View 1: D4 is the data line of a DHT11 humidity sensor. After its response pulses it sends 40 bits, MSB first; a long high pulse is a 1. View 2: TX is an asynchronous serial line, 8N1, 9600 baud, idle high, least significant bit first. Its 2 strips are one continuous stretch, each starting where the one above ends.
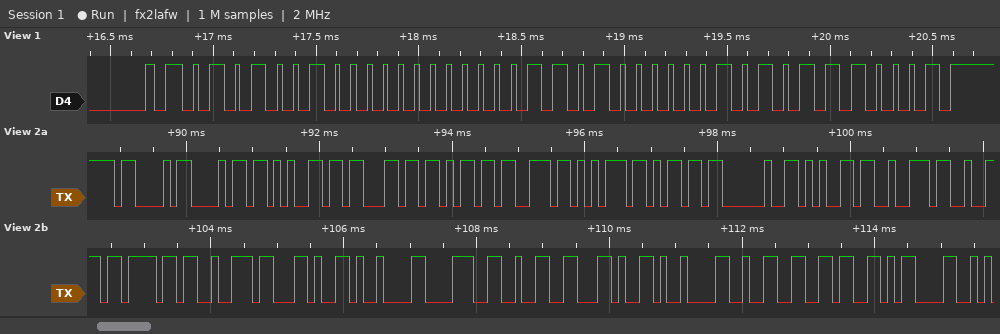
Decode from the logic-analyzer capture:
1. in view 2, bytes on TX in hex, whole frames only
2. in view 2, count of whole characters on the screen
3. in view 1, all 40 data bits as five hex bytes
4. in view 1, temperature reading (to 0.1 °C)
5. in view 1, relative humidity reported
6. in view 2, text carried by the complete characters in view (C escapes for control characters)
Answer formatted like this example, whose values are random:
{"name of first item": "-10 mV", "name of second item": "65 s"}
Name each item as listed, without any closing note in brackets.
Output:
{"in view 2, bytes on TX in hex, whole frames only": "43 68 65 63 6B 73 75 6D 20 65 72 72 6F 72 2C 09 38 32 2C 09 32 36 0D", "in view 2, count of whole characters on the screen": "23", "in view 1, all 40 data bits as five hex bytes": "52 00 1A 05 71", "in view 1, temperature reading": "26.5 °C", "in view 1, relative humidity reported": "82 %", "in view 2, text carried by the complete characters in view": "\"Checksum error,\\t82,\\t26\\r\""}
